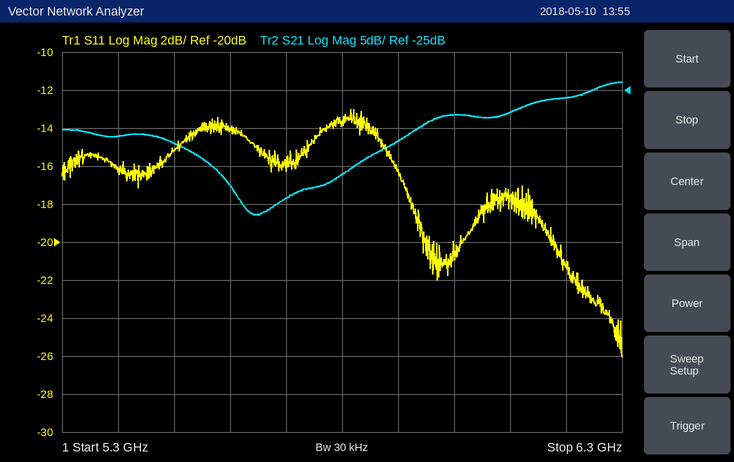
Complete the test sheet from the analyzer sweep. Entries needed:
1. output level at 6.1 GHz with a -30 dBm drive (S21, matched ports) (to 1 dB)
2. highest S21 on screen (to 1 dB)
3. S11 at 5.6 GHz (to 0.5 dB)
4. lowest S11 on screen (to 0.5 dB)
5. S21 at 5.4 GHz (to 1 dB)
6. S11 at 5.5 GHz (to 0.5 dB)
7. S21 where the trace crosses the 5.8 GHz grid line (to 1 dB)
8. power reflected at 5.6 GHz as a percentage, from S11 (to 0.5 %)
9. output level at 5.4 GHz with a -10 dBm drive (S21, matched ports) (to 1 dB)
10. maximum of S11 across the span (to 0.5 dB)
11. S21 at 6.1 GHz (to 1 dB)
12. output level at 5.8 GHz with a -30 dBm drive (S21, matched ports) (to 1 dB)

-58 dBm
-24 dB
-14.0 dB
-26.0 dB
-31 dB
-15.0 dB
-36 dB
4.0 %
-41 dBm
-13.0 dB
-28 dB
-66 dBm
